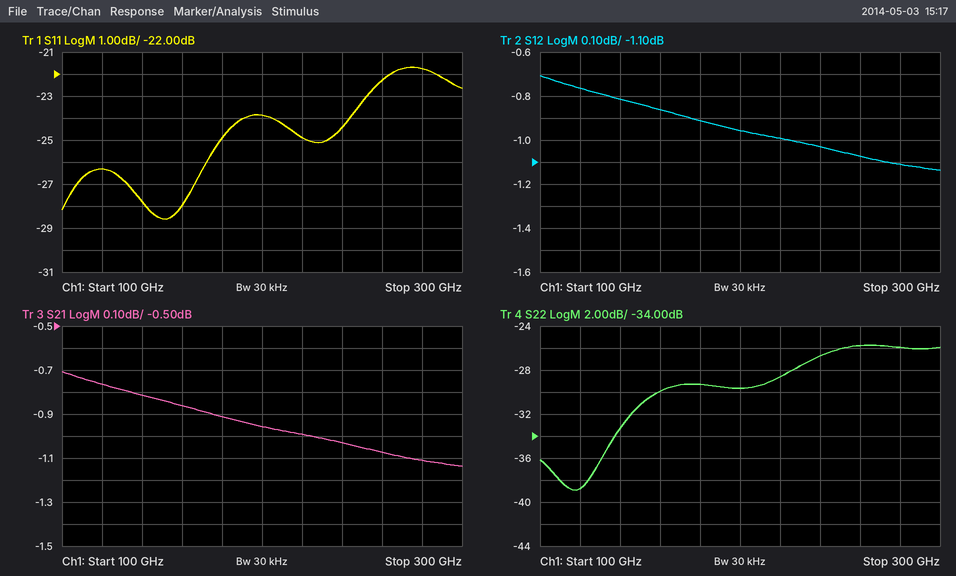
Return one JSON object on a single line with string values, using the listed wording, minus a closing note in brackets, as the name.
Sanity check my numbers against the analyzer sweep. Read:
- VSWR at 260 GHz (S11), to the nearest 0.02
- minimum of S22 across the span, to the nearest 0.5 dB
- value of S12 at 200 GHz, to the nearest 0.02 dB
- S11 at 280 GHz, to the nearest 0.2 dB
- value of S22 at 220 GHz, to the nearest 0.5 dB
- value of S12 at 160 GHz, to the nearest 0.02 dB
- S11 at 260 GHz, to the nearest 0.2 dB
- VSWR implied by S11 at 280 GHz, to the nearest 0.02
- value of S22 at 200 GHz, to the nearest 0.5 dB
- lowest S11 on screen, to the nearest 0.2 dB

{"VSWR at 260 GHz (S11), to the nearest 0.02": "1.16", "minimum of S22 across the span, to the nearest 0.5 dB": "-39.0 dB", "value of S12 at 200 GHz, to the nearest 0.02 dB": "-0.96 dB", "S11 at 280 GHz, to the nearest 0.2 dB": "-21.8 dB", "value of S22 at 220 GHz, to the nearest 0.5 dB": "-28.5 dB", "value of S12 at 160 GHz, to the nearest 0.02 dB": "-0.86 dB", "S11 at 260 GHz, to the nearest 0.2 dB": "-22.2 dB", "VSWR implied by S11 at 280 GHz, to the nearest 0.02": "1.18", "value of S22 at 200 GHz, to the nearest 0.5 dB": "-29.5 dB", "lowest S11 on screen, to the nearest 0.2 dB": "-28.6 dB"}
